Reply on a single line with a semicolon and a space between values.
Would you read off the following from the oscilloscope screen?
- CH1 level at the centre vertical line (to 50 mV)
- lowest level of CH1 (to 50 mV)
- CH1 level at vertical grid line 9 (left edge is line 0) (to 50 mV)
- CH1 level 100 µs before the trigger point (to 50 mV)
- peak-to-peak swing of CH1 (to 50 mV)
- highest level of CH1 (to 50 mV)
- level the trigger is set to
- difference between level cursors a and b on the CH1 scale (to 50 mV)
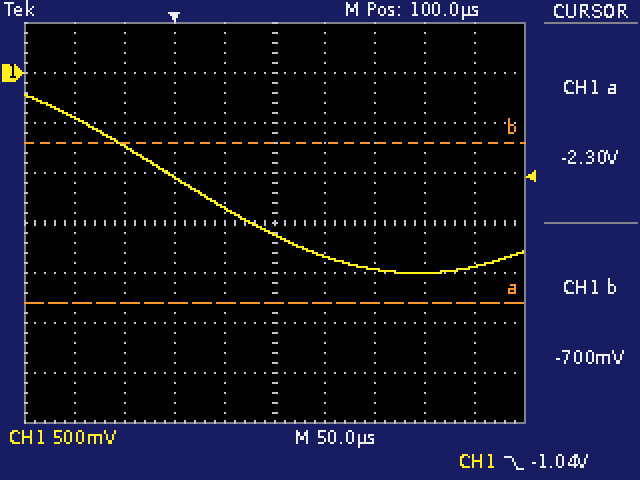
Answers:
-1.60 V; -2.00 V; -1.95 V; -450 mV; 1.80 V; -200 mV; -1.04 V; 1.60 V
